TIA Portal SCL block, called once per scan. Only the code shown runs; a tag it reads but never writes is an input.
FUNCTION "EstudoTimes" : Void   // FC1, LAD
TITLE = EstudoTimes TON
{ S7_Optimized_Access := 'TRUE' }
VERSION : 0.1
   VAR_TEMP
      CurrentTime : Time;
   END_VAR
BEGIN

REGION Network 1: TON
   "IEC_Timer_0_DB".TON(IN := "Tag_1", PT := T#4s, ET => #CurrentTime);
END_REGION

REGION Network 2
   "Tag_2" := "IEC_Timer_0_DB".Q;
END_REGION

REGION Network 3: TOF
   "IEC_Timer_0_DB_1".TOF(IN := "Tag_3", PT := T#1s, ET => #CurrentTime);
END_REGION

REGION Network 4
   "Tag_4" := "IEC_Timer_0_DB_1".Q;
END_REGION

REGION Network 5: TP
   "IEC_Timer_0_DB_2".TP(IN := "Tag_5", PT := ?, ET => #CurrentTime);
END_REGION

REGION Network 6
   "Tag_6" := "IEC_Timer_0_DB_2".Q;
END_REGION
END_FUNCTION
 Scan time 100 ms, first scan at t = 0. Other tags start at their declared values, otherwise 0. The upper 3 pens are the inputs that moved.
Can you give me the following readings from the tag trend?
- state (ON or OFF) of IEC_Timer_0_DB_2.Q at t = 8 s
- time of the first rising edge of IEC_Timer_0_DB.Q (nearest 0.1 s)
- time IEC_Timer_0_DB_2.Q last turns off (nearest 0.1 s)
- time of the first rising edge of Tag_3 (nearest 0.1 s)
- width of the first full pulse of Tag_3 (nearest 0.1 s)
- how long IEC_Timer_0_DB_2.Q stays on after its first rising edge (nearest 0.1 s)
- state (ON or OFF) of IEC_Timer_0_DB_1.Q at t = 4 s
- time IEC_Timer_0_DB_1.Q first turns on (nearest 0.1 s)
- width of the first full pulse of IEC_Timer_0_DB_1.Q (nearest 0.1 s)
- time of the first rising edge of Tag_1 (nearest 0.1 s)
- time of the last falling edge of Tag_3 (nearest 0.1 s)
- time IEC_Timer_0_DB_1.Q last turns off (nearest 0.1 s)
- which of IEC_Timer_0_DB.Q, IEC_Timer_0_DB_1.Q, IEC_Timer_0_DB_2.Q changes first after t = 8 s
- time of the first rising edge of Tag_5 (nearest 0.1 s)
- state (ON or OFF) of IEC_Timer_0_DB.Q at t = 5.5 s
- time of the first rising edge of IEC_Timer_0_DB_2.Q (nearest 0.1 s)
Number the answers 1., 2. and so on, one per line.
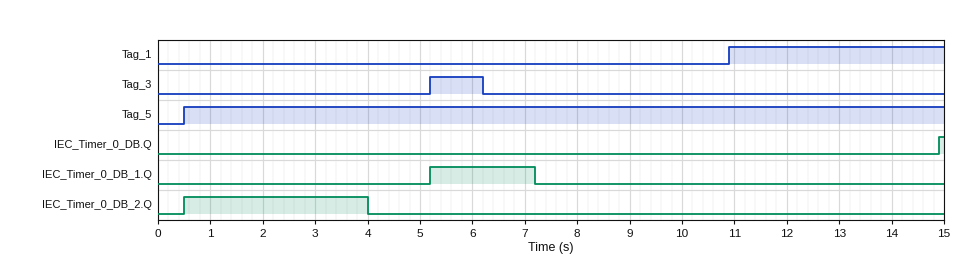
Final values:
1. OFF
2. 14.9 s
3. 4.0 s
4. 5.2 s
5. 1.0 s
6. 3.5 s
7. OFF
8. 5.2 s
9. 2.0 s
10. 10.9 s
11. 6.2 s
12. 7.2 s
13. IEC_Timer_0_DB.Q
14. 0.5 s
15. OFF
16. 0.5 s
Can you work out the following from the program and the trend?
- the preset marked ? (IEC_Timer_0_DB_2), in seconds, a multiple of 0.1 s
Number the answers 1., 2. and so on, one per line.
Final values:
1. 3.5 s
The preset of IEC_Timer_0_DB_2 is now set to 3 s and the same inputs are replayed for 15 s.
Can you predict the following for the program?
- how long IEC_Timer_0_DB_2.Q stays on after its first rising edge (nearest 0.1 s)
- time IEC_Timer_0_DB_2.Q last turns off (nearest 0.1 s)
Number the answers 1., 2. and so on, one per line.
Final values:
1. 3.0 s
2. 3.5 s
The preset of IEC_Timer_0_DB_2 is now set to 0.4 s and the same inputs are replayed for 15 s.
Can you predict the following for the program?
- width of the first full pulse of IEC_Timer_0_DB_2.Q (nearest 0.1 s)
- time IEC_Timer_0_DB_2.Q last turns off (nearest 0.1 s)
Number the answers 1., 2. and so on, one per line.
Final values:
1. 0.4 s
2. 0.9 s
